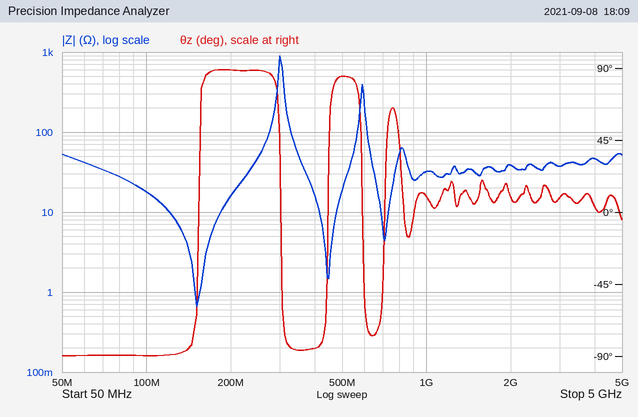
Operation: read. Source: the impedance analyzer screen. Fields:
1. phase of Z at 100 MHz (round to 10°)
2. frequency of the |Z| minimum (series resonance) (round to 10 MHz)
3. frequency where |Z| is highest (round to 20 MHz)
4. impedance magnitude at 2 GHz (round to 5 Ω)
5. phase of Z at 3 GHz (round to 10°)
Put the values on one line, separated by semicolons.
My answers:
-90°; 150 MHz; 300 MHz; 40 Ω; 10°
